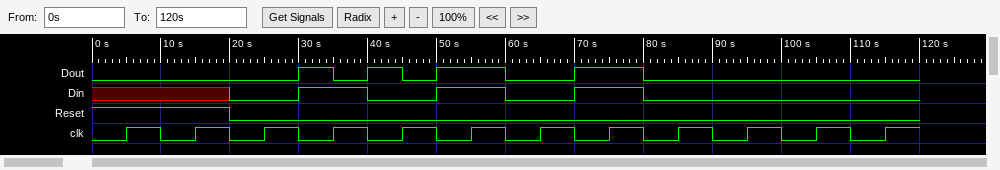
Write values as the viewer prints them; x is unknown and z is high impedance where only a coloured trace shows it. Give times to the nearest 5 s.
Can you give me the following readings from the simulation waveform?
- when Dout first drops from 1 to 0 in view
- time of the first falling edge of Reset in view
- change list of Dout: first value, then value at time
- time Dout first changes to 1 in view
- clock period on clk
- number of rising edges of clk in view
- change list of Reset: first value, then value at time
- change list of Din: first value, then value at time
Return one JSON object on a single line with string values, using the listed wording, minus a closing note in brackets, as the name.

{"when Dout first drops from 1 to 0 in view": "35 s", "time of the first falling edge of Reset in view": "20 s", "change list of Dout: first value, then value at time": "0, 1 at 30 s, 0 at 35 s, 1 at 40 s, 0 at 45 s, 1 at 50 s, 0 at 60 s, 1 at 70 s, 0 at 80 s", "time Dout first changes to 1 in view": "30 s", "clock period on clk": "10 s", "number of rising edges of clk in view": "12", "change list of Reset: first value, then value at time": "1, 0 at 20 s", "change list of Din: first value, then value at time": "x, 0 at 20 s, 1 at 30 s, 0 at 40 s, 1 at 50 s, 0 at 60 s, 1 at 70 s, 0 at 80 s"}
